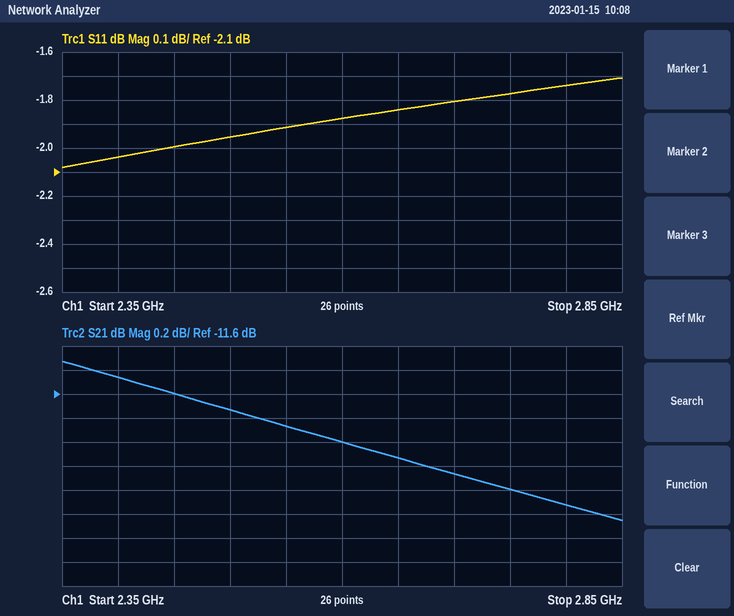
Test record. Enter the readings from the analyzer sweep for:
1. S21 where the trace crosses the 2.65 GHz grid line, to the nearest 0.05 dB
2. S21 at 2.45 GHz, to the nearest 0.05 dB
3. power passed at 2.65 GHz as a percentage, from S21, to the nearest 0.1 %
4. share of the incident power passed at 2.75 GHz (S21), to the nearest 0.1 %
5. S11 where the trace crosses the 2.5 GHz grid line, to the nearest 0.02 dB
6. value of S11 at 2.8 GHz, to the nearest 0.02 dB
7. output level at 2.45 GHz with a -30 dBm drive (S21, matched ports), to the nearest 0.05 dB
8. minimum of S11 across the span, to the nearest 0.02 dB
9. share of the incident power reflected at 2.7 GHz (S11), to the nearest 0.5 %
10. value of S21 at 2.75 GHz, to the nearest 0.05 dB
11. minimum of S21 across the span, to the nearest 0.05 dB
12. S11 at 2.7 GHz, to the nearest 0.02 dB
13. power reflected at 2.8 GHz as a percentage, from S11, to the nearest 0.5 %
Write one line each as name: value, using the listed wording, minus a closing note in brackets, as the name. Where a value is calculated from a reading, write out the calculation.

S21 where the trace crosses the 2.65 GHz grid line, to the nearest 0.05 dB: -12.15 dB
S21 at 2.45 GHz, to the nearest 0.05 dB: -11.60 dB
power passed at 2.65 GHz as a percentage, from S21, to the nearest 0.1 %: 10^(-12.15/10) ≈ 6.1 %
share of the incident power passed at 2.75 GHz (S21), to the nearest 0.1 %: 10^(-12.4/10) ≈ 5.8 %
S11 where the trace crosses the 2.5 GHz grid line, to the nearest 0.02 dB: -1.96 dB
value of S11 at 2.8 GHz, to the nearest 0.02 dB: -1.74 dB
output level at 2.45 GHz with a -30 dBm drive (S21, matched ports), to the nearest 0.05 dB: -30 dBm + (-11.60 dB) = -41.60 dBm
minimum of S11 across the span, to the nearest 0.02 dB: -2.08 dB
share of the incident power reflected at 2.7 GHz (S11), to the nearest 0.5 %: 10^(-1.8/10) ≈ 66.1 %, so 66.0 % to the nearest 0.5 %
value of S21 at 2.75 GHz, to the nearest 0.05 dB: -12.40 dB
minimum of S21 across the span, to the nearest 0.05 dB: -12.65 dB
S11 at 2.7 GHz, to the nearest 0.02 dB: -1.80 dB
power reflected at 2.8 GHz as a percentage, from S11, to the nearest 0.5 %: 10^(-1.74/10) ≈ 67.0 %
